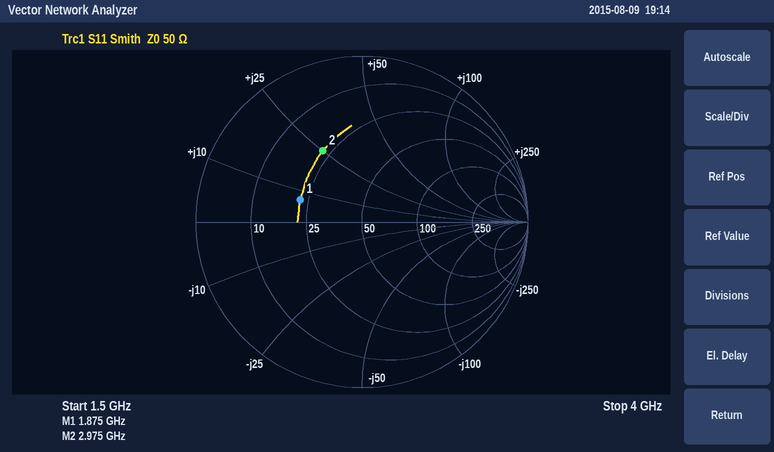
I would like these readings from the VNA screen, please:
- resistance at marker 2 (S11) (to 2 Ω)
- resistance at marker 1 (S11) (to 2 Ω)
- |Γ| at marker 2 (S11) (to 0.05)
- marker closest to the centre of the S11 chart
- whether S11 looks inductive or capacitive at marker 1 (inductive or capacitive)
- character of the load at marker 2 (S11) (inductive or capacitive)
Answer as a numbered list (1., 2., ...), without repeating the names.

1. 22 Ω
2. 22 Ω
3. 0.50
4. marker 1
5. inductive
6. inductive
